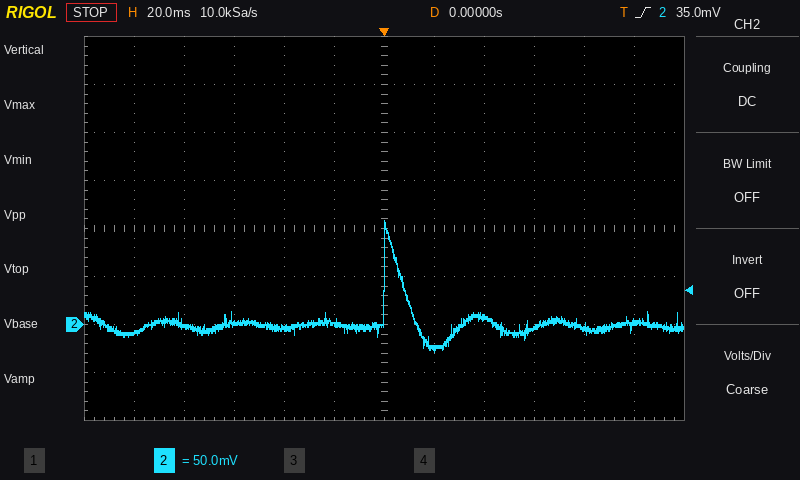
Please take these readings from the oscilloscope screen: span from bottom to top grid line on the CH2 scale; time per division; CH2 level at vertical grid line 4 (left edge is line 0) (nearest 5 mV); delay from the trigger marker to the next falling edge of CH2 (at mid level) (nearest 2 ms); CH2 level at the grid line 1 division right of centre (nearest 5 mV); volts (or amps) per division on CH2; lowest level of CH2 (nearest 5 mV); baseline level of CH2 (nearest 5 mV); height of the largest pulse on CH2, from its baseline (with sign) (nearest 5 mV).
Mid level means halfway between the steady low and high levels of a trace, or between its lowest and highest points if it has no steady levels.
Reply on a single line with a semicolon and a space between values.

400 mV; 20 ms; -5 mV; 8 ms; -25 mV; 50 mV; -30 mV; 0 mV; +110 mV
